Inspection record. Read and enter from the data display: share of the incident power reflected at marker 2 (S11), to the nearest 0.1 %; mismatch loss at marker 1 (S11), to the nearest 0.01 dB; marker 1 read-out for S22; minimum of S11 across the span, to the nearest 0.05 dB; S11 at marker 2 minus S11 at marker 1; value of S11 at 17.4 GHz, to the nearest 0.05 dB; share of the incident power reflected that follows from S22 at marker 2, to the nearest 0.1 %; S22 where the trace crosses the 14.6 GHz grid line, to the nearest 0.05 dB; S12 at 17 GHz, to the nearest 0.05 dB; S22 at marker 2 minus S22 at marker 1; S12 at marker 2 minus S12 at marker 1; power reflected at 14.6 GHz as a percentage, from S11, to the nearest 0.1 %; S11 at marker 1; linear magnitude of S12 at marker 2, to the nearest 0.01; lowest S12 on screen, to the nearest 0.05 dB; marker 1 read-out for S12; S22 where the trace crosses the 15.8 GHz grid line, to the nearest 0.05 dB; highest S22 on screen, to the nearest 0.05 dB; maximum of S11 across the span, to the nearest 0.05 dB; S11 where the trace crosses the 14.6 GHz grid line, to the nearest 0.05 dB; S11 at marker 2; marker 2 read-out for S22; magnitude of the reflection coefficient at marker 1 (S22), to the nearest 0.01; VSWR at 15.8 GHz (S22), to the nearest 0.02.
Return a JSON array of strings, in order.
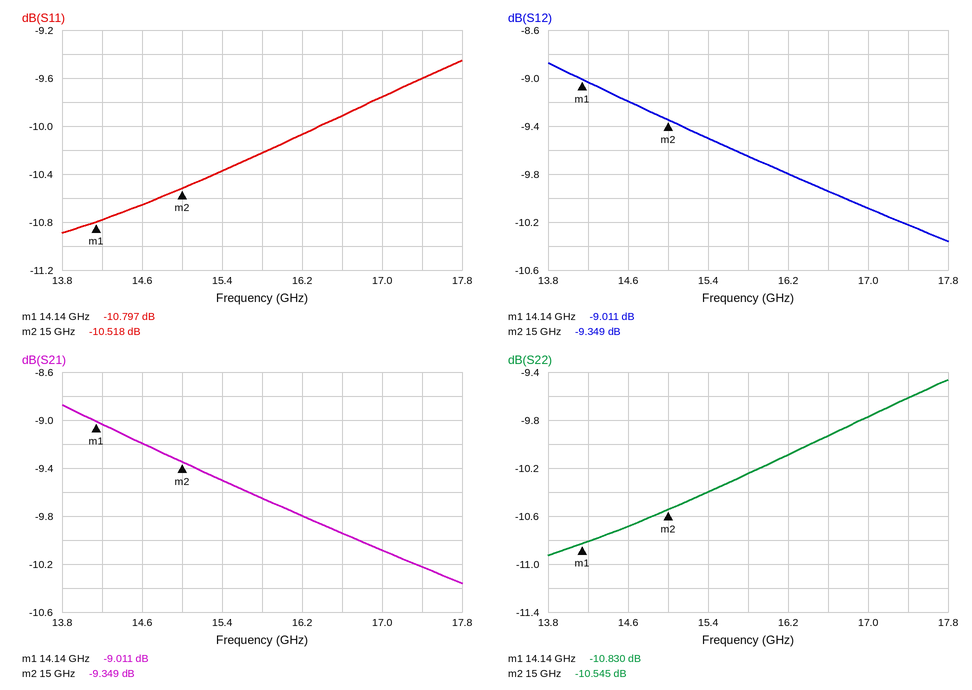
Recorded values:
["8.9 %", "0.38 dB", "-10.830 dB", "-10.90 dB", "0.279 dB", "-9.60 dB", "8.8 %", "-10.70 dB", "-10.10 dB", "0.285 dB", "-0.338 dB", "8.6 %", "-10.797 dB", "0.34", "-10.35 dB", "-9.011 dB", "-10.25 dB", "-9.45 dB", "-9.45 dB", "-10.65 dB", "-10.518 dB", "-10.545 dB", "0.29", "1.88"]
